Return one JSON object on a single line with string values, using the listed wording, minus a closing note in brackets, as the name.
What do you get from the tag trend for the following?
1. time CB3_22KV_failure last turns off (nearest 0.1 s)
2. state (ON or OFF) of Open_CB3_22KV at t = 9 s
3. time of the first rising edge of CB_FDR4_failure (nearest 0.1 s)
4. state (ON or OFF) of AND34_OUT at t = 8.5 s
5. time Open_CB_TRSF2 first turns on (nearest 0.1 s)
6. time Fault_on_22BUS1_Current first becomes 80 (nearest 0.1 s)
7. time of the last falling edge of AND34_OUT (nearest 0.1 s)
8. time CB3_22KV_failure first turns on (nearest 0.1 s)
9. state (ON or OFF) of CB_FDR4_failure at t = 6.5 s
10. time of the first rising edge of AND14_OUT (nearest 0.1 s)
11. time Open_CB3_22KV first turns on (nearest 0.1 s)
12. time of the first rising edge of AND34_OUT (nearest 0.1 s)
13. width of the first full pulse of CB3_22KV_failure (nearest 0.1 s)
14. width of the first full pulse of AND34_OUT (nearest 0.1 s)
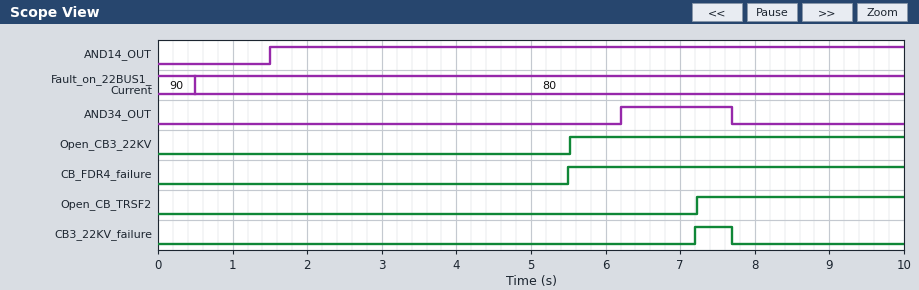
{"time CB3_22KV_failure last turns off": "7.7 s", "state (ON or OFF) of Open_CB3_22KV at t = 9 s": "ON", "time of the first rising edge of CB_FDR4_failure": "5.5 s", "state (ON or OFF) of AND34_OUT at t = 8.5 s": "OFF", "time Open_CB_TRSF2 first turns on": "7.2 s", "time Fault_on_22BUS1_Current first becomes 80": "0.5 s", "time of the last falling edge of AND34_OUT": "7.7 s", "time CB3_22KV_failure first turns on": "7.2 s", "state (ON or OFF) of CB_FDR4_failure at t = 6.5 s": "ON", "time of the first rising edge of AND14_OUT": "1.5 s", "time Open_CB3_22KV first turns on": "5.5 s", "time of the first rising edge of AND34_OUT": "6.2 s", "width of the first full pulse of CB3_22KV_failure": "0.5 s", "width of the first full pulse of AND34_OUT": "1.5 s"}
